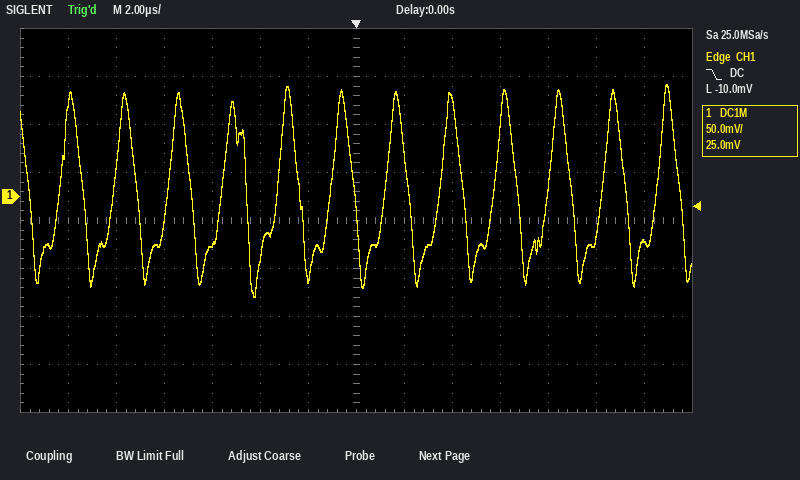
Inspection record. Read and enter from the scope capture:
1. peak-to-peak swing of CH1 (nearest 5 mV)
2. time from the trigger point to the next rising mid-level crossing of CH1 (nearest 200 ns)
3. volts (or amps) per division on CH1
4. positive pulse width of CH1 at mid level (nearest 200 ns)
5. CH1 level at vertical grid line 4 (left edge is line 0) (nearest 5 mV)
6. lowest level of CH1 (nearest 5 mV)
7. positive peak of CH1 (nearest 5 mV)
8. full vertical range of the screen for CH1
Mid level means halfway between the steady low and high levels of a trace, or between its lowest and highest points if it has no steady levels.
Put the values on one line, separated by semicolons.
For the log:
220 mV; 1.2 µs; 50 mV; 1.0 µs; -50 mV; -105 mV; 115 mV; 400 mV
